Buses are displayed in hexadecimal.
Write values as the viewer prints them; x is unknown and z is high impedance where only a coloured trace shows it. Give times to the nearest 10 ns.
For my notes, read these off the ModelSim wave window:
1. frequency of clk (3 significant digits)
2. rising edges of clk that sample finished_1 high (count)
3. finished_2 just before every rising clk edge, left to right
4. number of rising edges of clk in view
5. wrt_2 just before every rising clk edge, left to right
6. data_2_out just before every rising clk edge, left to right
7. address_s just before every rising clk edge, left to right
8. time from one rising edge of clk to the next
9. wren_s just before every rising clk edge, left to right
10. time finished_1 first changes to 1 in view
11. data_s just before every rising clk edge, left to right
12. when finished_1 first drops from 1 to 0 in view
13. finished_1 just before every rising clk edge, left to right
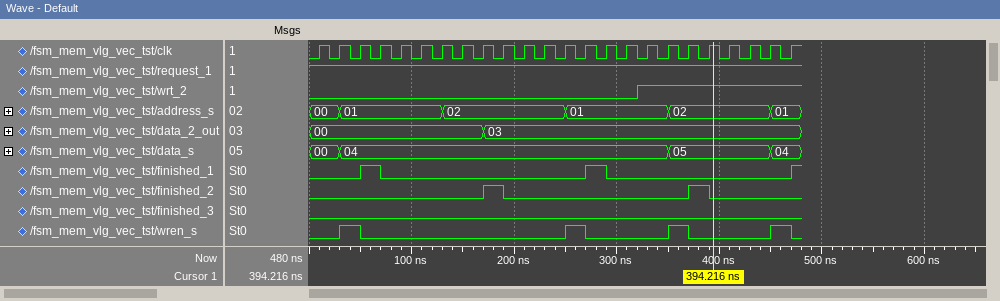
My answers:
50.0 MHz
2
0 0 0 0 0 0 0 0 0 1 0 0 0 0 0 0 0 0 0 1 0 0 0 0
24
0 0 0 0 0 0 0 0 0 0 0 0 0 0 0 0 1 1 1 1 1 1 1 1
00, 00, 00, 00, 00, 00, 00, 00, 00, 03, 03, 03, 03, 03, 03, 03, 03, 03, 03, 03, 03, 03, 03, 03
00, 00, 01, 01, 01, 01, 01, 02, 02, 02, 02, 02, 02, 01, 01, 01, 01, 01, 02, 02, 02, 02, 02, 01
20 ns
0 0 1 0 0 0 0 0 0 0 0 0 0 1 0 0 0 0 1 0 0 0 0 1
50 ns
00, 00, 04, 04, 04, 04, 04, 04, 04, 04, 04, 04, 04, 04, 04, 04, 04, 04, 05, 05, 05, 05, 05, 04
70 ns
0 0 0 1 0 0 0 0 0 0 0 0 0 0 1 0 0 0 0 0 0 0 0 0
